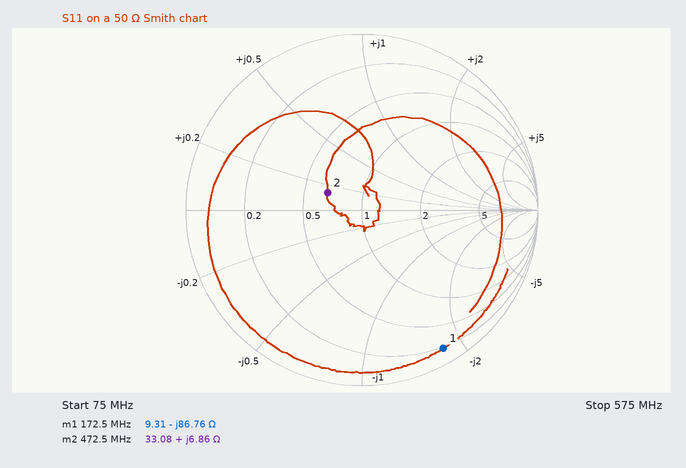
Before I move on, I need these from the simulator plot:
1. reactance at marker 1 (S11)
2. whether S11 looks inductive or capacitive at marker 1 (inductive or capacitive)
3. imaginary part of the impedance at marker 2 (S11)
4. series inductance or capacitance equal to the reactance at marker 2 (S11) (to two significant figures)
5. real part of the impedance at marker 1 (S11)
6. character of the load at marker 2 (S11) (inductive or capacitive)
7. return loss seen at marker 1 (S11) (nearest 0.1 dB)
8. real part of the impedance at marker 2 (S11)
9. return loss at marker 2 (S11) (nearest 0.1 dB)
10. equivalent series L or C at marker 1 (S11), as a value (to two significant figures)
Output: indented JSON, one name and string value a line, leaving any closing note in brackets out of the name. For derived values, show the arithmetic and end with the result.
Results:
{
  "reactance at marker 1": "-86.76 Ω",
  "whether S11 looks inductive or capacitive at marker 1": "capacitive",
  "imaginary part of the impedance at marker 2": "+6.86 Ω",
  "series inductance or capacitance equal to the reactance at marker 2 (S11)": "L = 6.86 Ω/(2π × 472.5 MHz) ≈ 2.3 nH",
  "real part of the impedance at marker 1": "9.31 Ω",
  "character of the load at marker 2 (S11)": "inductive",
  "return loss seen at marker 1 (S11)": "0.8 dB",
  "real part of the impedance at marker 2": "33.08 Ω",
  "return loss at marker 2 (S11)": "13.2 dB",
  "equivalent series L or C at marker 1 (S11), as a value": "C = 1/(2π × 172.5 MHz × 86.76 Ω) ≈ 11 pF"
}
